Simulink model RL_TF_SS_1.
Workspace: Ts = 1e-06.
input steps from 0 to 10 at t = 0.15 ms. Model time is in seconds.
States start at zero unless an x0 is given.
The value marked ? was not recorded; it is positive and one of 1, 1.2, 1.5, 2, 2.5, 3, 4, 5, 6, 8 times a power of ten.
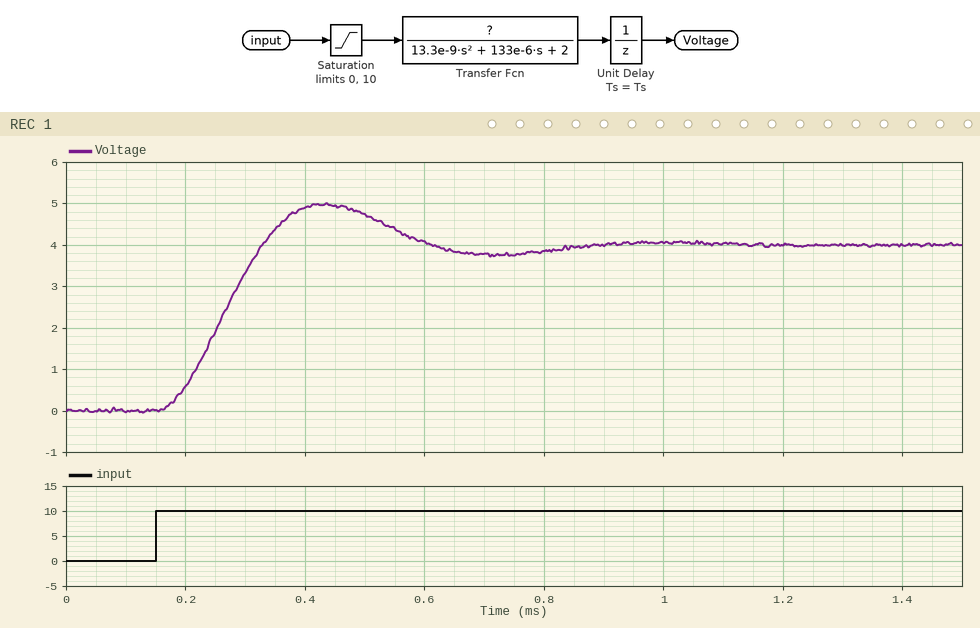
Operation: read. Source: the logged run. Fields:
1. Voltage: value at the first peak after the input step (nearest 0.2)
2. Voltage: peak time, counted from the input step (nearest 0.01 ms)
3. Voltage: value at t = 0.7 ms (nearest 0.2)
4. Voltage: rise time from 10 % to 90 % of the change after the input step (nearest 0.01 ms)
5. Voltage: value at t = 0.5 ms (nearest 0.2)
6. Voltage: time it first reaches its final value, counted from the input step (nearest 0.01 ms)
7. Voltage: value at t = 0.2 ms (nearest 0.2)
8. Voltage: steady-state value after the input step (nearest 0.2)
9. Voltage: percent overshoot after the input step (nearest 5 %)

5.0
0.28 ms
3.8
0.12 ms
4.8
0.18 ms
0.6
4.0
25 %
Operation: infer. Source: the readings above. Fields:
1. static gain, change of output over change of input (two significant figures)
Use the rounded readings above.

0.40
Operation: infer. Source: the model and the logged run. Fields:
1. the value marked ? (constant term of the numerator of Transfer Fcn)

0.8
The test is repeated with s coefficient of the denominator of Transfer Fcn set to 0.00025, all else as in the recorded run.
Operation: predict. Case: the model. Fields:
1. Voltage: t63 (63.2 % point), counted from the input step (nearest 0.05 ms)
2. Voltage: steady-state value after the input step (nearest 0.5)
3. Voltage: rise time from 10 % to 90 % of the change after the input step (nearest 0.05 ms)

0.15 ms
4.0
0.20 ms
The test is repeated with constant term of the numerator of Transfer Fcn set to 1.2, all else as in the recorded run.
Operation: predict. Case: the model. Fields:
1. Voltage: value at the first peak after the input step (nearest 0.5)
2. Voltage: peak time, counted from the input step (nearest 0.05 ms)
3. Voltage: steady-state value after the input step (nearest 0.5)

7.5
0.30 ms
6.0
